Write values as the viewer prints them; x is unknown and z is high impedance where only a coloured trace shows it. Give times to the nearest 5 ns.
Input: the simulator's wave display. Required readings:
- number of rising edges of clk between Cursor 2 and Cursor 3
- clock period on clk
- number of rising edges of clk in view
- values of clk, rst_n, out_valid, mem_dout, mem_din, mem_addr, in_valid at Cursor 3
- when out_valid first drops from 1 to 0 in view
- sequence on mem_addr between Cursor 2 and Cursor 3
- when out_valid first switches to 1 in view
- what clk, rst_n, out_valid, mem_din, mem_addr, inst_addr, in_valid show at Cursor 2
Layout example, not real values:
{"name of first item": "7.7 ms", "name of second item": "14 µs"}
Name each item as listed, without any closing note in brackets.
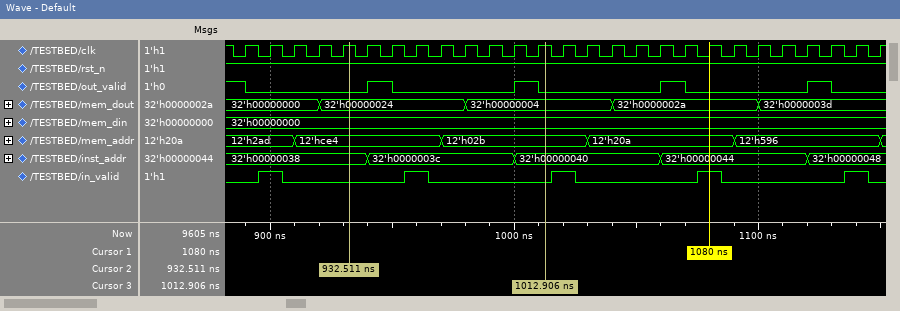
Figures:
{"number of rising edges of clk between Cursor 2 and Cursor 3": "8", "clock period on clk": "10 ns", "number of rising edges of clk in view": "27", "values of clk, rst_n, out_valid, mem_dout, mem_din, mem_addr, in_valid at Cursor 3": "clk=1, rst_n=1, out_valid=0, mem_dout=32'h00000004, mem_din=32'h00000000, mem_addr=12'h02b, in_valid=0", "when out_valid first drops from 1 to 0 in view": "890 ns", "sequence on mem_addr between Cursor 2 and Cursor 3": "12'hce4, 12'h02b", "when out_valid first switches to 1 in view": "940 ns", "what clk, rst_n, out_valid, mem_din, mem_addr, inst_addr, in_valid show at Cursor 2": "clk=1, rst_n=1, out_valid=0, mem_din=32'h00000000, mem_addr=12'hce4, inst_addr=32'h00000038, in_valid=0"}
